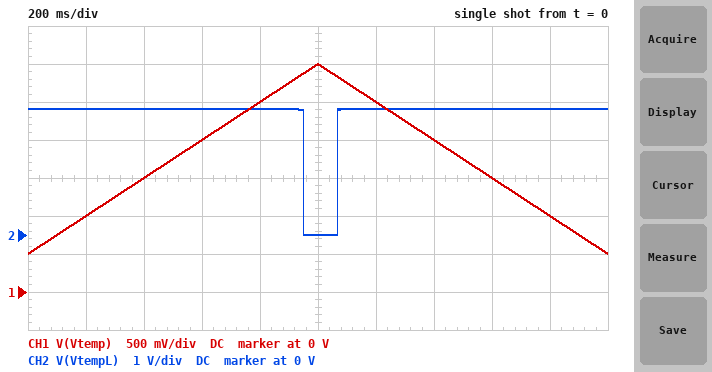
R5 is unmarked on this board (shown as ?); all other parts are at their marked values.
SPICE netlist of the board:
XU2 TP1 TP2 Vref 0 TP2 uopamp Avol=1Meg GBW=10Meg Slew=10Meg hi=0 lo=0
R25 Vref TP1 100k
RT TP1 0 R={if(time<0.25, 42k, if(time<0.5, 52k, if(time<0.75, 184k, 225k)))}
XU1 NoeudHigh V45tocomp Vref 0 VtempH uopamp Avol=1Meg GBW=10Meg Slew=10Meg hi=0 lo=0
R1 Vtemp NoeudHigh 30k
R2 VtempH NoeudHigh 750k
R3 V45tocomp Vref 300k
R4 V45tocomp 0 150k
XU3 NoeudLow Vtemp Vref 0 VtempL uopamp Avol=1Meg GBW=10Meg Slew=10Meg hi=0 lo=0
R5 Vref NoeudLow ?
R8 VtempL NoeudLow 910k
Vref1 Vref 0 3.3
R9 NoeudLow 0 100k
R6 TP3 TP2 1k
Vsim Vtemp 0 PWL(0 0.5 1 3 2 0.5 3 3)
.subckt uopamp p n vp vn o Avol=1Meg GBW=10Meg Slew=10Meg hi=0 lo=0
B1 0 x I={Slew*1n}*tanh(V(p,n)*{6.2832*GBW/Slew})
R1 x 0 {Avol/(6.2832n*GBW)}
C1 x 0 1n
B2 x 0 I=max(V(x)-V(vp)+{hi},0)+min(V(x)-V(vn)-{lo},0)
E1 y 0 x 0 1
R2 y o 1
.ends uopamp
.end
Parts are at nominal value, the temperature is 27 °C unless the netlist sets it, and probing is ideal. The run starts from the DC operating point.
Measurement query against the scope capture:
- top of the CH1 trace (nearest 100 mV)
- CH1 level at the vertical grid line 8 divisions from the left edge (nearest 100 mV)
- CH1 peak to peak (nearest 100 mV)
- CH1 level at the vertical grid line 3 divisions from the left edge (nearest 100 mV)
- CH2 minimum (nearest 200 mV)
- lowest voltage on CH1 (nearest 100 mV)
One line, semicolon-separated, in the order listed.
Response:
3.0 V; 1.5 V; 2.5 V; 2.0 V; 0 V; 500 mV
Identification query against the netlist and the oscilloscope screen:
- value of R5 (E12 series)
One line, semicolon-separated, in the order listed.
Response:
15 kΩ
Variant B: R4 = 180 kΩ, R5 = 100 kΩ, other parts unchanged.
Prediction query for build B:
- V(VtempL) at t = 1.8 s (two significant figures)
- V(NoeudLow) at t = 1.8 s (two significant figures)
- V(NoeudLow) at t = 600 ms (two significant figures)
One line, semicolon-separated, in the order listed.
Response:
3.3 V; 1.7 V; 1.6 V
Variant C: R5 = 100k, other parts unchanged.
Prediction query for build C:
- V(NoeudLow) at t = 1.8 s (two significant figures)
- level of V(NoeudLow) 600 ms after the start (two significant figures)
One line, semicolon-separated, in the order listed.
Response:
1.7 V; 1.6 V
